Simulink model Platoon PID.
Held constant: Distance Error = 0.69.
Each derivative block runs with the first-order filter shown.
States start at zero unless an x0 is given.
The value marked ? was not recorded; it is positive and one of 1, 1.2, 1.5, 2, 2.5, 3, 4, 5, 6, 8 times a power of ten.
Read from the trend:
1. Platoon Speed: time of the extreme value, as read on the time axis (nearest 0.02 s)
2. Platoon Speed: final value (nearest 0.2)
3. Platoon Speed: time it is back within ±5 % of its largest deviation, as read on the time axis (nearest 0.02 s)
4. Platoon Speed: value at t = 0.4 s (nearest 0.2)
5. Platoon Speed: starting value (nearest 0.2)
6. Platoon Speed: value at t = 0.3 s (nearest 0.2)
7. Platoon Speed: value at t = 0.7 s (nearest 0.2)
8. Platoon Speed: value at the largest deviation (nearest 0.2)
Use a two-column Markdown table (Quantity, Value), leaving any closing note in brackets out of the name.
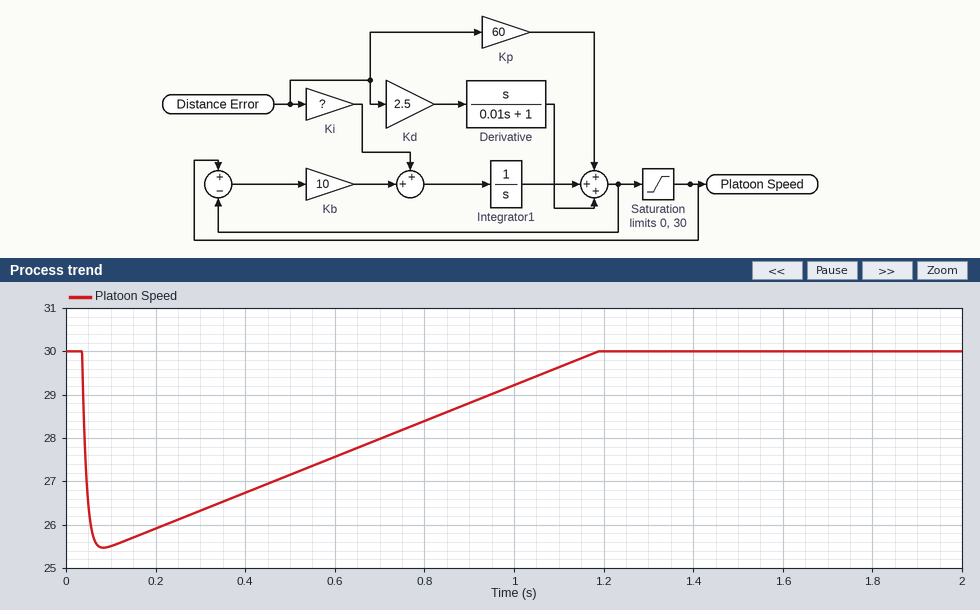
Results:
| Quantity | Value |
|---|---|
| Platoon Speed: time of the extreme value, as read on the time axis | 0.08 s |
| Platoon Speed: final value | 30.0 |
| Platoon Speed: time it is back within ±5 % of its largest deviation, as read on the time axis | 1.14 s |
| Platoon Speed: value at t = 0.4 s | 26.8 |
| Platoon Speed: starting value | 30.0 |
| Platoon Speed: value at t = 0.3 s | 26.4 |
| Platoon Speed: value at t = 0.7 s | 28.0 |
| Platoon Speed: value at the largest deviation | 25.4 |
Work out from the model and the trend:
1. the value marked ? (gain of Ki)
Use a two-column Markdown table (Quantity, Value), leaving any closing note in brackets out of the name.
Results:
| Quantity | Value |
|---|---|
| the value marked ? | 6 |
